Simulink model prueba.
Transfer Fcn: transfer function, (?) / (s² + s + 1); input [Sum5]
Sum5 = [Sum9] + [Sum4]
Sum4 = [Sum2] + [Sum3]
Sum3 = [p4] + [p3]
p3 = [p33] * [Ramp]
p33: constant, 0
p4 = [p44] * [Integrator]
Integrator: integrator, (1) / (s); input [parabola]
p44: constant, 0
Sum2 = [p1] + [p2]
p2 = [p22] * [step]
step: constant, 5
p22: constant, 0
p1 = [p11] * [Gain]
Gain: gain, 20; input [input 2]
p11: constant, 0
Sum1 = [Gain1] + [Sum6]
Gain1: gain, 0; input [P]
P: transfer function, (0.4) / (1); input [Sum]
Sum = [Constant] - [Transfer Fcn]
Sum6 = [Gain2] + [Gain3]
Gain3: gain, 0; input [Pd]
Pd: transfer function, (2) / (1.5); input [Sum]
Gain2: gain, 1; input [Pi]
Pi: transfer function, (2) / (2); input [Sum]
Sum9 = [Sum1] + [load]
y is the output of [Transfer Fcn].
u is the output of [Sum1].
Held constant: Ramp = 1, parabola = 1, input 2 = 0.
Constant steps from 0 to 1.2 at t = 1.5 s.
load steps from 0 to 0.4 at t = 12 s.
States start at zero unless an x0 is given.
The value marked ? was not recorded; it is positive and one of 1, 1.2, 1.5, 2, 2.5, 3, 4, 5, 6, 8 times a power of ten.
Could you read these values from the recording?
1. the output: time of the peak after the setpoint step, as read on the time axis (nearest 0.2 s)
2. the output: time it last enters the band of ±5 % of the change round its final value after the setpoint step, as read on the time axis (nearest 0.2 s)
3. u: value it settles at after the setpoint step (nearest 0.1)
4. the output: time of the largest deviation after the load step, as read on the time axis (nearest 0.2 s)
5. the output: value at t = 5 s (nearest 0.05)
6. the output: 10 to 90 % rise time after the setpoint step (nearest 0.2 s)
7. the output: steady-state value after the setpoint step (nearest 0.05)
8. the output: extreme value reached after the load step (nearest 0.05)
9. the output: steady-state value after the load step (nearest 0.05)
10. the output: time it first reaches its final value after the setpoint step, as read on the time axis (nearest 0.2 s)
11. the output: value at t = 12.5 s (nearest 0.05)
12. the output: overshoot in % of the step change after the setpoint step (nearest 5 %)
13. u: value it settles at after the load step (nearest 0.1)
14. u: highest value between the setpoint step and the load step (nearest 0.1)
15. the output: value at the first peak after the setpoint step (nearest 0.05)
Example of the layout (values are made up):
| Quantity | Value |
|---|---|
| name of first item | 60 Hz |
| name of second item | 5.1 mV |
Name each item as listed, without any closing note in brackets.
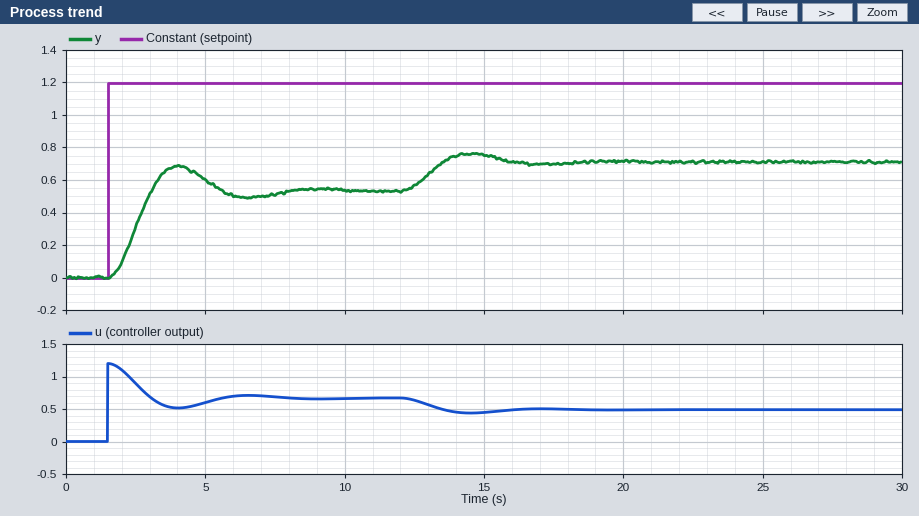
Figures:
| Quantity | Value |
|---|---|
| the output: time of the peak after the setpoint step, as read on the time axis | 4.0 s |
| the output: time it last enters the band of ±5 % of the change round its final value after the setpoint step, as read on the time axis | 7.4 s |
| u: value it settles at after the setpoint step | 0.7 |
| the output: time of the largest deviation after the load step, as read on the time axis | 14.6 s |
| the output: value at t = 5 s | 0.60 |
| the output: 10 to 90 % rise time after the setpoint step | 1.0 s |
| the output: steady-state value after the setpoint step | 0.55 |
| the output: extreme value reached after the load step | 0.75 |
| the output: steady-state value after the load step | 0.70 |
| the output: time it first reaches its final value after the setpoint step, as read on the time axis | 3.0 s |
| the output: value at t = 12.5 s | 0.55 |
| the output: overshoot in % of the step change after the setpoint step | 30 % |
| u: value it settles at after the load step | 0.5 |
| u: highest value between the setpoint step and the load step | 1.2 |
| the output: value at the first peak after the setpoint step | 0.70 |
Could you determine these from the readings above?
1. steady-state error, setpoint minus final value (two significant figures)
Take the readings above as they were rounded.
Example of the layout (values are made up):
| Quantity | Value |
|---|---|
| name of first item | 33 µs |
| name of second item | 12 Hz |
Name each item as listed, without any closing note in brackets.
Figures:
| Quantity | Value |
|---|---|
| steady-state error, setpoint minus final value | 0.65 |
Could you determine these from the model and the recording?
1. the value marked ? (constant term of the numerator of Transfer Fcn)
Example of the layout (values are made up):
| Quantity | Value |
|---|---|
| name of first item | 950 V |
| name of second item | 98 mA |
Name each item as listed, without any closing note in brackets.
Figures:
| Quantity | Value |
|---|---|
| the value marked ? | 0.8 |
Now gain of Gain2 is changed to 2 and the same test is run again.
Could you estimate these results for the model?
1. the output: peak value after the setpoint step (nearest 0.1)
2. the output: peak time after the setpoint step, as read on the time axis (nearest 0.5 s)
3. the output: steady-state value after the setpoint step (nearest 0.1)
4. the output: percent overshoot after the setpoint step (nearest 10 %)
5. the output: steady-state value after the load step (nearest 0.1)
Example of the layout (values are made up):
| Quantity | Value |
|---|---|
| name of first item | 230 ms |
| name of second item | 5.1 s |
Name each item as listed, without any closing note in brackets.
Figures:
| Quantity | Value |
|---|---|
| the output: peak value after the setpoint step | 1.0 |
| the output: peak time after the setpoint step, as read on the time axis | 3.5 s |
| the output: steady-state value after the setpoint step | 0.7 |
| the output: percent overshoot after the setpoint step | 40 % |
| the output: steady-state value after the load step | 0.9 |
